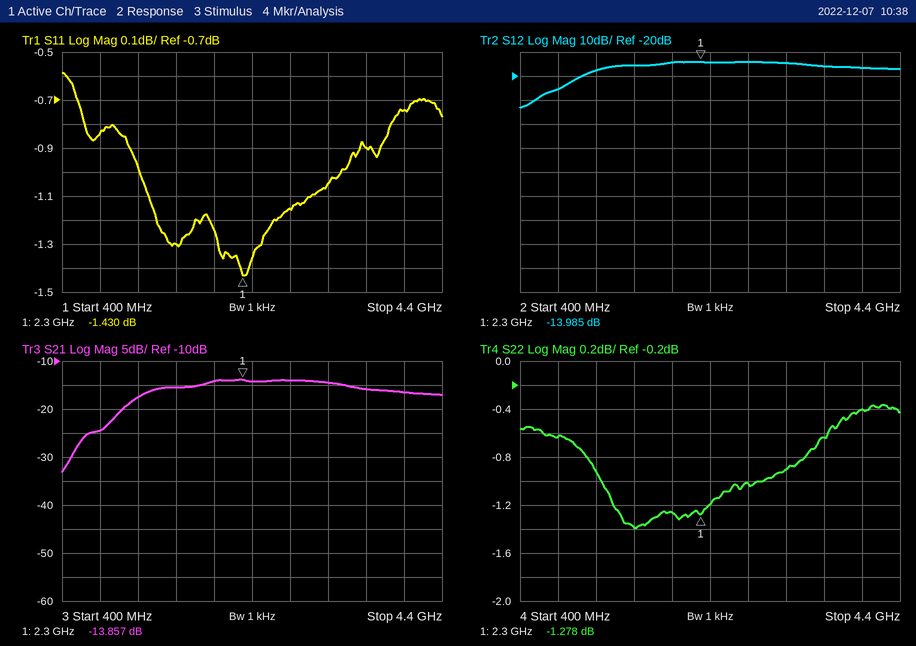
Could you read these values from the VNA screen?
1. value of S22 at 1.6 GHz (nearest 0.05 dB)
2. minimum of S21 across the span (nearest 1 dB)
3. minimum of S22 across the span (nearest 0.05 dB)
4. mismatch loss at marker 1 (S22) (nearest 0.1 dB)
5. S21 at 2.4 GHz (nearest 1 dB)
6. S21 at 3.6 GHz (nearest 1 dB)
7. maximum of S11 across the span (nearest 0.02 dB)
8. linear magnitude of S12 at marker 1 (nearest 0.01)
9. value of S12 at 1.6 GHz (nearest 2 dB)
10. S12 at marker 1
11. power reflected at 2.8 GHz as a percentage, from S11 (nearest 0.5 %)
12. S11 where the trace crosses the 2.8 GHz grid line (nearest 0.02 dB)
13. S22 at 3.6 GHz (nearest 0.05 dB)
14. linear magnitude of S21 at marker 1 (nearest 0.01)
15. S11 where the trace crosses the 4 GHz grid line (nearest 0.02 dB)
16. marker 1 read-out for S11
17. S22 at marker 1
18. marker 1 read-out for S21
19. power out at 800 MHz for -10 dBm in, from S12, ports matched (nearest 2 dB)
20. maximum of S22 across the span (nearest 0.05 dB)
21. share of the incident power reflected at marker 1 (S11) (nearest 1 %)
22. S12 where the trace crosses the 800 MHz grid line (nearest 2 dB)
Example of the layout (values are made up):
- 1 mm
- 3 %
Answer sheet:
- -1.40 dB
- -33 dB
- -1.40 dB
- 5.9 dB
- -14 dB
- -16 dB
- -0.58 dB
- 0.20
- -16 dB
- -13.985 dB
- 76.5 %
- -1.16 dB
- -0.65 dB
- 0.20
- -0.74 dB
- -1.430 dB
- -1.278 dB
- -13.857 dB
- -36 dBm
- -0.35 dB
- 72 %
- -26 dB
